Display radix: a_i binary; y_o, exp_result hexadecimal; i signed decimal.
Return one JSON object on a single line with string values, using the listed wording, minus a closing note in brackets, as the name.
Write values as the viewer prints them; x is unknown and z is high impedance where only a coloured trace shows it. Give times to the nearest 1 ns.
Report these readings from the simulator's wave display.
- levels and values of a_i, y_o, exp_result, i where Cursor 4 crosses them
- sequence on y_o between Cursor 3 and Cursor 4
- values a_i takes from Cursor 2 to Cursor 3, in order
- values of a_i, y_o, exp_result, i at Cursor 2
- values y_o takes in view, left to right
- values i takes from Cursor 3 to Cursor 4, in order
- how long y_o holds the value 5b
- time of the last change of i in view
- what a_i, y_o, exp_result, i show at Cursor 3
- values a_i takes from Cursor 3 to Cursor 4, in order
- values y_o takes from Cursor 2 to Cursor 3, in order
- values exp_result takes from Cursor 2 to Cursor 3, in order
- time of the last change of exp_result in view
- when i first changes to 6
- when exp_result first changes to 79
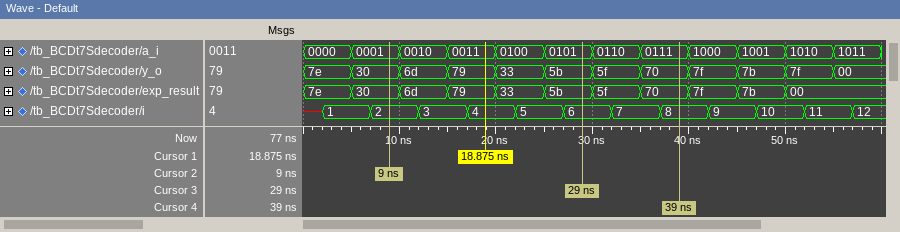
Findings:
{"levels and values of a_i, y_o, exp_result, i where Cursor 4 crosses them": "a_i=0111, y_o=70, exp_result=70, i=8", "sequence on y_o between Cursor 3 and Cursor 4": "5b, 5f, 70", "values a_i takes from Cursor 2 to Cursor 3, in order": "0001, 0010, 0011, 0100, 0101", "values of a_i, y_o, exp_result, i at Cursor 2": "a_i=0001, y_o=30, exp_result=30, i=2", "values y_o takes in view, left to right": "7e, 30, 6d, 79, 33, 5b, 5f, 70, 7f, 7b, 7f, 00", "values i takes from Cursor 3 to Cursor 4, in order": "6, 7, 8", "how long y_o holds the value 5b": "5 ns", "time of the last change of i in view": "57 ns", "what a_i, y_o, exp_result, i show at Cursor 3": "a_i=0101, y_o=5b, exp_result=5b, i=6", "values a_i takes from Cursor 3 to Cursor 4, in order": "0101, 0110, 0111", "values y_o takes from Cursor 2 to Cursor 3, in order": "30, 6d, 79, 33, 5b", "values exp_result takes from Cursor 2 to Cursor 3, in order": "30, 6d, 79, 33, 5b", "time of the last change of exp_result in view": "50 ns", "when i first changes to 6": "27 ns", "when exp_result first changes to 79": "15 ns"}
